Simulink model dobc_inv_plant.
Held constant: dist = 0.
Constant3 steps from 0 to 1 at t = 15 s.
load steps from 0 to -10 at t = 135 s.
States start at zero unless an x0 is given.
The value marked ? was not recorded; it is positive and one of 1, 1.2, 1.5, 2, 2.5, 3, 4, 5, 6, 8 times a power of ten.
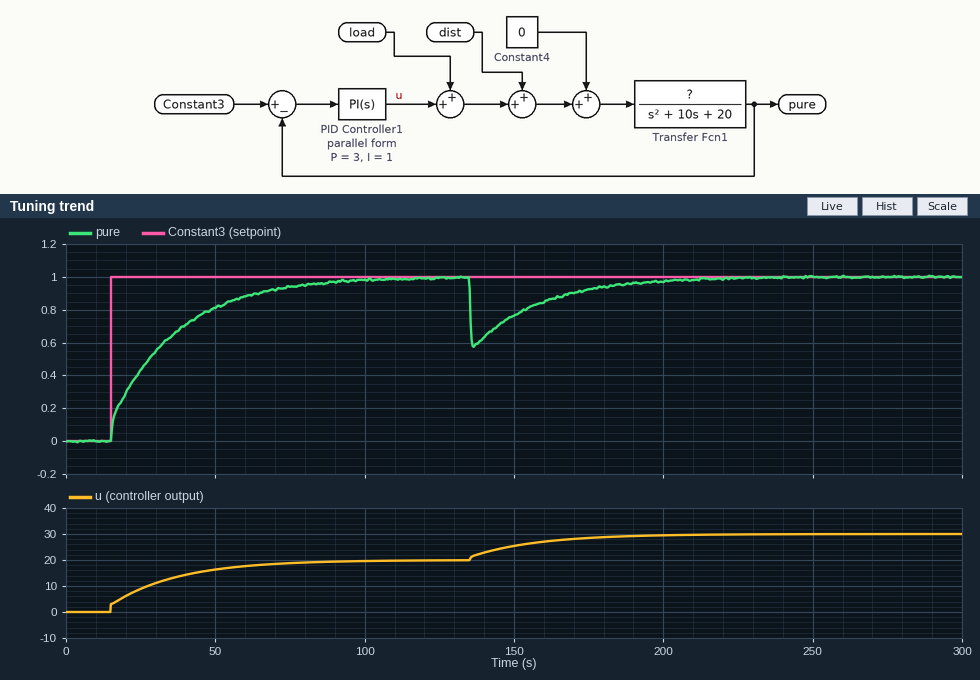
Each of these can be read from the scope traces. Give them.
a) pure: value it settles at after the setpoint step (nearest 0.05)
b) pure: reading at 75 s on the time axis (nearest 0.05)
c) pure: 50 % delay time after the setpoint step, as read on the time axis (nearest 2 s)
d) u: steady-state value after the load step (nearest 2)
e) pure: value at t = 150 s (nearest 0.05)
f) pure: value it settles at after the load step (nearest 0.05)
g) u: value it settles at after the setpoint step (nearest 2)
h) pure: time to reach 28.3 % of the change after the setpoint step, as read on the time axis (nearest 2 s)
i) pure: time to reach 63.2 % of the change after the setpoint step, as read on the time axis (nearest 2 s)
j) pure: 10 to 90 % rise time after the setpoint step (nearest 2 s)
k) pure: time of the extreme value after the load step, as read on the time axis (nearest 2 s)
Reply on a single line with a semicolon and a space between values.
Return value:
1.00; 0.95; 28 s; 30; 0.75; 1.00; 20; 20 s; 34 s; 48 s; 136 s
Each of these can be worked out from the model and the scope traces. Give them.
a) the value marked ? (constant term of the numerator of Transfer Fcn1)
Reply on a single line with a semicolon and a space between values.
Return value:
1
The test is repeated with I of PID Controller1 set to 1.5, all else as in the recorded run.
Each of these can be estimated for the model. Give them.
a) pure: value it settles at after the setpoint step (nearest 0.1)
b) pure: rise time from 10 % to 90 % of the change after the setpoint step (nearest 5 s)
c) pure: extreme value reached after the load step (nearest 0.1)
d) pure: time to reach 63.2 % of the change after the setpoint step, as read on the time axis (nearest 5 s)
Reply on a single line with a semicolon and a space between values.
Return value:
1.0; 30 s; 0.6; 30 s
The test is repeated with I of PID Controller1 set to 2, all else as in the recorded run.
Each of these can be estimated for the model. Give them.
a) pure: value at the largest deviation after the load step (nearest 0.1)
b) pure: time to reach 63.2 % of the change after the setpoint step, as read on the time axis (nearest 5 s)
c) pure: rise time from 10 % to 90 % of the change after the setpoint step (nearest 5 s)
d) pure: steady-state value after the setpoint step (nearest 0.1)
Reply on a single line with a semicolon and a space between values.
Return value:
0.6; 25 s; 25 s; 1.0
